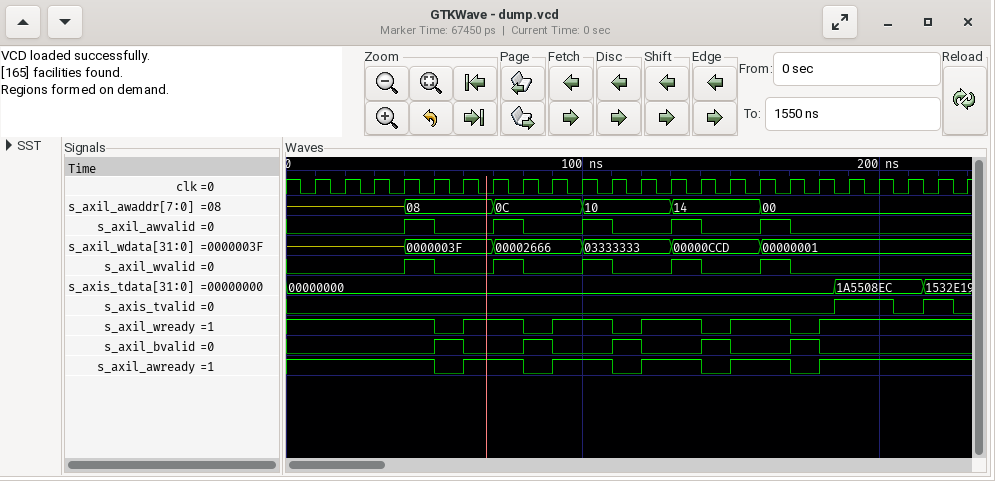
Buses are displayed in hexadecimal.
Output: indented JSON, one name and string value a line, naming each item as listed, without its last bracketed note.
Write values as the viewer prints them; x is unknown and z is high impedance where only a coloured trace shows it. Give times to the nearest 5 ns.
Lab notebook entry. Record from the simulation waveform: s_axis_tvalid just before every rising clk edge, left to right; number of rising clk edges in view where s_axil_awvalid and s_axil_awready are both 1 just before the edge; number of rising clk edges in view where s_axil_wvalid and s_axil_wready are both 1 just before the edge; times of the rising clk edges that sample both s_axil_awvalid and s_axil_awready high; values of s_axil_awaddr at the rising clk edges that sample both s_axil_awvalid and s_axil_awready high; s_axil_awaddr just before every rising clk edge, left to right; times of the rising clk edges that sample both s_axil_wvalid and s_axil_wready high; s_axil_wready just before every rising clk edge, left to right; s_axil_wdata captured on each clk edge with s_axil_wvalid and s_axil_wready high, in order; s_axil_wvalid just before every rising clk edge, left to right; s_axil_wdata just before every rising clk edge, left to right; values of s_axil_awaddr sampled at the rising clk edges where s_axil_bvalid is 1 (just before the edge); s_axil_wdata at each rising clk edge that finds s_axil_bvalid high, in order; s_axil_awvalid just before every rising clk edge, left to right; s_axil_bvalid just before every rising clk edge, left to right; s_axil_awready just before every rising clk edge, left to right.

{
  "s_axis_tvalid just before every rising clk edge, left to right": "0 0 0 0 0 0 0 0 0 0 0 0 0 0 0 0 0 0 1 1 0 1 0",
  "number of rising clk edges in view where s_axil_awvalid and s_axil_awready are both 1 just before the edge": "5",
  "number of rising clk edges in view where s_axil_wvalid and s_axil_wready are both 1 just before the edge": "5",
  "times of the rising clk edges that sample both s_axil_awvalid and s_axil_awready high": "50 ns, 80 ns, 110 ns, 140 ns, 170 ns",
  "values of s_axil_awaddr at the rising clk edges that sample both s_axil_awvalid and s_axil_awready high": "08, 0C, 10, 14, 00",
  "s_axil_awaddr just before every rising clk edge, left to right": "z, z, z, z, 08, 08, 08, 0C, 0C, 0C, 10, 10, 10, 14, 14, 14, 00, 00, 00, 00, 00, 00, 00",
  "times of the rising clk edges that sample both s_axil_wvalid and s_axil_wready high": "50 ns, 80 ns, 110 ns, 140 ns, 170 ns",
  "s_axil_wready just before every rising clk edge, left to right": "1 1 1 1 1 0 1 1 0 1 1 0 1 1 0 1 1 0 1 1 1 1 1",
  "s_axil_wdata captured on each clk edge with s_axil_wvalid and s_axil_wready high, in order": "0000003F, 00002666, 03333333, 00000CCD, 00000001",
  "s_axil_wvalid just before every rising clk edge, left to right": "0 0 0 0 1 0 0 1 0 0 1 0 0 1 0 0 1 0 0 0 0 0 0",
  "s_axil_wdata just before every rising clk edge, left to right": "z, z, z, z, 0000003F, 0000003F, 0000003F, 00002666, 00002666, 00002666, 03333333, 03333333, 03333333, 00000CCD, 00000CCD, 00000CCD, 00000001, 00000001, 00000001, 00000001, 00000001, 00000001, 00000001",
  "values of s_axil_awaddr sampled at the rising clk edges where s_axil_bvalid is 1": "08, 0C, 10, 14, 00",
  "s_axil_wdata at each rising clk edge that finds s_axil_bvalid high, in order": "0000003F, 00002666, 03333333, 00000CCD, 00000001",
  "s_axil_awvalid just before every rising clk edge, left to right": "0 0 0 0 1 0 0 1 0 0 1 0 0 1 0 0 1 0 0 0 0 0 0",
  "s_axil_bvalid just before every rising clk edge, left to right": "0 0 0 0 0 1 0 0 1 0 0 1 0 0 1 0 0 1 0 0 0 0 0",
  "s_axil_awready just before every rising clk edge, left to right": "1 1 1 1 1 0 1 1 0 1 1 0 1 1 0 1 1 0 1 1 1 1 1"
}
